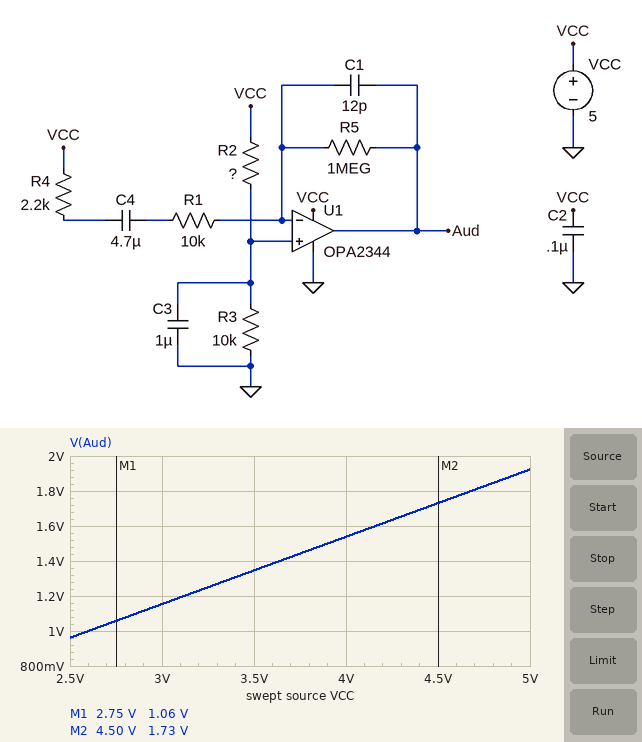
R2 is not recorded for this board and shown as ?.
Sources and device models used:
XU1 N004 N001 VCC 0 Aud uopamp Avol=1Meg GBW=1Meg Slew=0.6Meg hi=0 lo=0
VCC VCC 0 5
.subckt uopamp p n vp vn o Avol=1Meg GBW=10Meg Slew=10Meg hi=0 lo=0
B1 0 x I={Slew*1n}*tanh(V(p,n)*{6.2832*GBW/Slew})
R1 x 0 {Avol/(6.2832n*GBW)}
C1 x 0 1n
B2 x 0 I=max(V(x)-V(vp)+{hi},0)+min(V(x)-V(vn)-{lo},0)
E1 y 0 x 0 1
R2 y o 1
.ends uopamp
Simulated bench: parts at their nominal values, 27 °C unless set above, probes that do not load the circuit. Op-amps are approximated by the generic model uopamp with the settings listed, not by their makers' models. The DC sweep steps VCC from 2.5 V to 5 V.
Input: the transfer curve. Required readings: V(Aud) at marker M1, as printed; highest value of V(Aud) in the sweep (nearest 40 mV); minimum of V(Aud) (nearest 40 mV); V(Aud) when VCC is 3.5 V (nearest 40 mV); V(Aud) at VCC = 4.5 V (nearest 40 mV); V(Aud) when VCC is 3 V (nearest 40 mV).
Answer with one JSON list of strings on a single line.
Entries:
["1.06 V", "1.92 V", "960 mV", "1.36 V", "1.72 V", "1.16 V"]
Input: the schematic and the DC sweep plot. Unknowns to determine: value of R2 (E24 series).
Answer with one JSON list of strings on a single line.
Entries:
["16 kΩ"]
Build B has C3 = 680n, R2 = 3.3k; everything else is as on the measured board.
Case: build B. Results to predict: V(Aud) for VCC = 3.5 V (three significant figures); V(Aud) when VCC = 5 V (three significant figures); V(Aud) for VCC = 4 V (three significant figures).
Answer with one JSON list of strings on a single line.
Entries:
["2.63 V", "3.76 V", "3.01 V"]
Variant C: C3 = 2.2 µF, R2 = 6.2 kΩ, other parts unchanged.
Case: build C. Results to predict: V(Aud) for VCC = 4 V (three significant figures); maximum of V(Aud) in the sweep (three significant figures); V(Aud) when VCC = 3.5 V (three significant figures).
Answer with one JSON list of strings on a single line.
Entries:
["2.47 V", "3.09 V", "2.16 V"]
